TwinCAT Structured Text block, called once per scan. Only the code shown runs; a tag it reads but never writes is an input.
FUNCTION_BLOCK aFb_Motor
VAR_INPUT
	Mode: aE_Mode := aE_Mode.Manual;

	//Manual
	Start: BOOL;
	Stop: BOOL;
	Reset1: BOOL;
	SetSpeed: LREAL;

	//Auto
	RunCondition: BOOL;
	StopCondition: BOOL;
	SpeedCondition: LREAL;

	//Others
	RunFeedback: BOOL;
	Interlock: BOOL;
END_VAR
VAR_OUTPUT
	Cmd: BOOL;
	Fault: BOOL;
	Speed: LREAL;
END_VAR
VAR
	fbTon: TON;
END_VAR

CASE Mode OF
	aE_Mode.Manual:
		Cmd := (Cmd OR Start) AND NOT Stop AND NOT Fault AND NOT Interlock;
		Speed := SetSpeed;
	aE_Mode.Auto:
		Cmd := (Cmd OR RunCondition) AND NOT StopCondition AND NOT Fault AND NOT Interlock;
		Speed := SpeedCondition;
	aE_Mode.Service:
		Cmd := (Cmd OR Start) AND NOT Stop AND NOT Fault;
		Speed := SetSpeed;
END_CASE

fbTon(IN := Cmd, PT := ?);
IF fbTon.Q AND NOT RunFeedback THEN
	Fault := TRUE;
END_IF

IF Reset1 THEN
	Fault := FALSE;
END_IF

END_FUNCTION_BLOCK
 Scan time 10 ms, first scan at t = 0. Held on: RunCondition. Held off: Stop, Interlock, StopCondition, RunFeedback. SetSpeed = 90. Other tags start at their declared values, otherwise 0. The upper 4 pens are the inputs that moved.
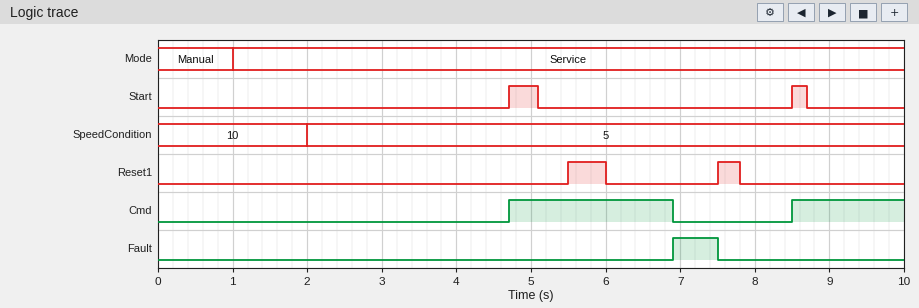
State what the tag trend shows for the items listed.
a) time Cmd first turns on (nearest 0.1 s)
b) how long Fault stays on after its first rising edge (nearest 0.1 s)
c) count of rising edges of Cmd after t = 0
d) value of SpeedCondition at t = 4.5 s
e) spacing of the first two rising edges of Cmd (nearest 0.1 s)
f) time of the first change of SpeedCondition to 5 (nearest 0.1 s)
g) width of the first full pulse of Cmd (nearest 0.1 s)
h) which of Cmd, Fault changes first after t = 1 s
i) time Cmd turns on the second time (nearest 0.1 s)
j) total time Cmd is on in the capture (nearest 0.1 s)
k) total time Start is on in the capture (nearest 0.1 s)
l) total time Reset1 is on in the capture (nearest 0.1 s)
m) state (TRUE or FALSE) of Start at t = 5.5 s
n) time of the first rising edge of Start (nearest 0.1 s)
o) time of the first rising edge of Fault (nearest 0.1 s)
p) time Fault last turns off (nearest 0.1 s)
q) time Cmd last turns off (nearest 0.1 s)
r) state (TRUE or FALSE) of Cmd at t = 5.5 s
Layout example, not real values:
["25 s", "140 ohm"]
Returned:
["4.7 s", "0.6 s", "2", "5", "3.8 s", "2.0 s", "2.2 s", "Cmd", "8.5 s", "3.7 s", "0.6 s", "0.8 s", "FALSE", "4.7 s", "6.9 s", "7.5 s", "6.9 s", "TRUE"]
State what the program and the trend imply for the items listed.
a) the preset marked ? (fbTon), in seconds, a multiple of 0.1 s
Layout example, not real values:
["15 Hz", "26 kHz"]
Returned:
["2.2 s"]
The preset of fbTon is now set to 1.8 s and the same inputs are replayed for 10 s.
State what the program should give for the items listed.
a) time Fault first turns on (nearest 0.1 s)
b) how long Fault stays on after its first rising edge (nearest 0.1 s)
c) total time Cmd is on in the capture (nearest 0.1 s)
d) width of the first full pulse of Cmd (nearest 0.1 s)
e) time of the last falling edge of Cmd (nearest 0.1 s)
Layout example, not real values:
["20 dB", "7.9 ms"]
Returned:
["6.5 s", "1.0 s", "3.3 s", "1.8 s", "6.5 s"]
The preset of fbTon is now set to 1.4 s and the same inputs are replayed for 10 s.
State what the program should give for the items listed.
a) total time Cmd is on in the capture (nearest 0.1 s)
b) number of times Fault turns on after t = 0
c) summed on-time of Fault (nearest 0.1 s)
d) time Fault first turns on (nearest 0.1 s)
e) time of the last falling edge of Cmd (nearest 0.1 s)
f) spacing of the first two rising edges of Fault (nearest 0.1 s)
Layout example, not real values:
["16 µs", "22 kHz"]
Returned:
["2.8 s", "2", "1.5 s", "6.1 s", "9.9 s", "3.8 s"]
